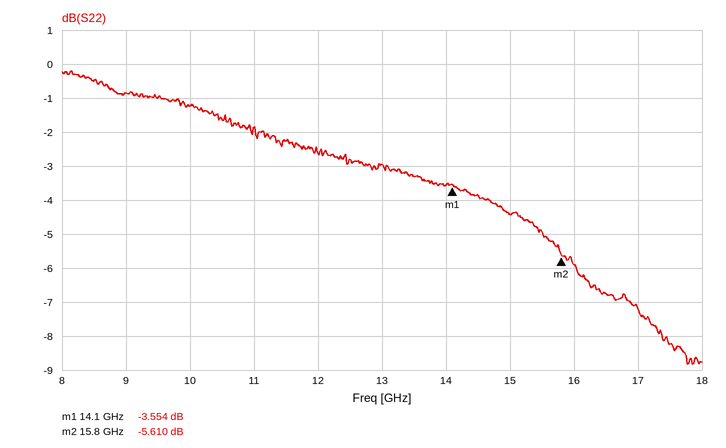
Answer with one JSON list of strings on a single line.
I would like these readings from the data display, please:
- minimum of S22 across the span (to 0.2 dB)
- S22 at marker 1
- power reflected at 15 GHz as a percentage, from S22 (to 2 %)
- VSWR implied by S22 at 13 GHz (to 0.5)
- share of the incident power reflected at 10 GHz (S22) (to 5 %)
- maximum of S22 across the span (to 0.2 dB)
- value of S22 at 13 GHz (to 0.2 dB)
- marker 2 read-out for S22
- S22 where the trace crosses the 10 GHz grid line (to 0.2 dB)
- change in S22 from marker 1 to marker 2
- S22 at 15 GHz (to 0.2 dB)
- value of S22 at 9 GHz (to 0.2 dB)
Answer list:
["-8.8 dB", "-3.554 dB", "36 %", "6.0", "75 %", "-0.2 dB", "-3.0 dB", "-5.610 dB", "-1.2 dB", "-2.056 dB", "-4.4 dB", "-0.8 dB"]
